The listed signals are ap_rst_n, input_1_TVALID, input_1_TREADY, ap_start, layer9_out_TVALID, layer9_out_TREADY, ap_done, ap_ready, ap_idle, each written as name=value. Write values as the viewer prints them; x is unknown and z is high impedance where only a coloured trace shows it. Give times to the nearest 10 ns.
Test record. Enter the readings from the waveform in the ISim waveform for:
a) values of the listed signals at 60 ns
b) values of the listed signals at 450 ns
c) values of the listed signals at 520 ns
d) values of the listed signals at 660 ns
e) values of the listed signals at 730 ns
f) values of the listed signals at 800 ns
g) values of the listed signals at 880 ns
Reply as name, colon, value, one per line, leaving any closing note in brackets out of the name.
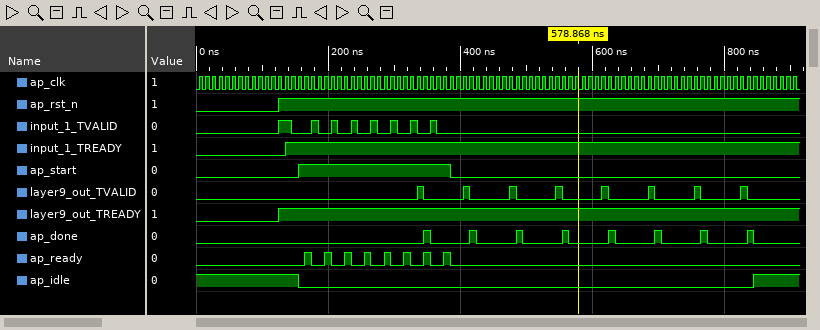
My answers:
values of the listed signals at 60 ns: ap_rst_n=0, input_1_TVALID=0, input_1_TREADY=0, ap_start=0, layer9_out_TVALID=0, layer9_out_TREADY=0, ap_done=0, ap_ready=0, ap_idle=1
values of the listed signals at 450 ns: ap_rst_n=1, input_1_TVALID=0, input_1_TREADY=1, ap_start=0, layer9_out_TVALID=0, layer9_out_TREADY=1, ap_done=0, ap_ready=0, ap_idle=0
values of the listed signals at 520 ns: ap_rst_n=1, input_1_TVALID=0, input_1_TREADY=1, ap_start=0, layer9_out_TVALID=0, layer9_out_TREADY=1, ap_done=0, ap_ready=0, ap_idle=0
values of the listed signals at 660 ns: ap_rst_n=1, input_1_TVALID=0, input_1_TREADY=1, ap_start=0, layer9_out_TVALID=0, layer9_out_TREADY=1, ap_done=0, ap_ready=0, ap_idle=0
values of the listed signals at 730 ns: ap_rst_n=1, input_1_TVALID=0, input_1_TREADY=1, ap_start=0, layer9_out_TVALID=0, layer9_out_TREADY=1, ap_done=0, ap_ready=0, ap_idle=0
values of the listed signals at 800 ns: ap_rst_n=1, input_1_TVALID=0, input_1_TREADY=1, ap_start=0, layer9_out_TVALID=0, layer9_out_TREADY=1, ap_done=0, ap_ready=0, ap_idle=0
values of the listed signals at 880 ns: ap_rst_n=1, input_1_TVALID=0, input_1_TREADY=1, ap_start=0, layer9_out_TVALID=0, layer9_out_TREADY=1, ap_done=0, ap_ready=0, ap_idle=1
